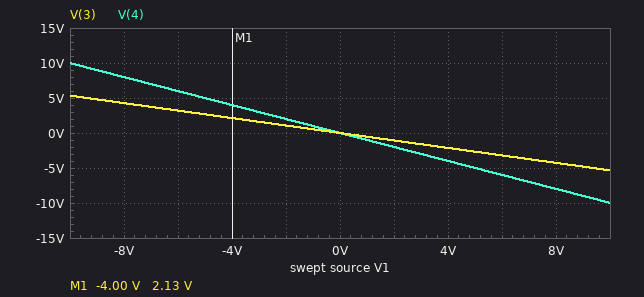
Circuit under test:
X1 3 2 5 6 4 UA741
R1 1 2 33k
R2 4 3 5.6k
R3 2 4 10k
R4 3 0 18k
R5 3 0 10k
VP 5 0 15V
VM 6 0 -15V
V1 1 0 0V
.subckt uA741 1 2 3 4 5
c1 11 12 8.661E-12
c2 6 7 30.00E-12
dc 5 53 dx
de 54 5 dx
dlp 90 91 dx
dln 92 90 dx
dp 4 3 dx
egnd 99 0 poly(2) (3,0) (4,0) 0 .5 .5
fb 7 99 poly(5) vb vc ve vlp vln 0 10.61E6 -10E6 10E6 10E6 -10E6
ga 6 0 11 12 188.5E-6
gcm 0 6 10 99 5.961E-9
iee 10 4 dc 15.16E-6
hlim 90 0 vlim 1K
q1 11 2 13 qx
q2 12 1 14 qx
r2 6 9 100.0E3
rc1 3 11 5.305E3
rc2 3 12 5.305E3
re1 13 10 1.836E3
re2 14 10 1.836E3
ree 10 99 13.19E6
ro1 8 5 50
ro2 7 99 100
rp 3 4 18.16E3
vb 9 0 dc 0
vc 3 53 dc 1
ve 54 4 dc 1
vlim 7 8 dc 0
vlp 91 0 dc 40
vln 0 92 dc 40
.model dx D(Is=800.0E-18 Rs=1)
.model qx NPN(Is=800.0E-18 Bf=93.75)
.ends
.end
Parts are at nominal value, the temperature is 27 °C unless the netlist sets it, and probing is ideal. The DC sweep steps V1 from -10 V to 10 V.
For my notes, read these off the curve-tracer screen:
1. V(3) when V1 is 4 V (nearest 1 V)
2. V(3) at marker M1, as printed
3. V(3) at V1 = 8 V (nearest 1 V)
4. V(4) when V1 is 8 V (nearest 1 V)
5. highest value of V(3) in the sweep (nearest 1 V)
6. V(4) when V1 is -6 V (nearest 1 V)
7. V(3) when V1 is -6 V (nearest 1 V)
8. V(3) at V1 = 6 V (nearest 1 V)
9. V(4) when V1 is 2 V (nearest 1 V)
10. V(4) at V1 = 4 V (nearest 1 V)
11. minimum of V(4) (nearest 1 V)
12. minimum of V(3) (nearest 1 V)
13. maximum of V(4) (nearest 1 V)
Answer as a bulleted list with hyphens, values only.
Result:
- -2 V
- 2.13 V
- -4 V
- -8 V
- 5 V
- 6 V
- 3 V
- -3 V
- -2 V
- -4 V
- -10 V
- -5 V
- 10 V
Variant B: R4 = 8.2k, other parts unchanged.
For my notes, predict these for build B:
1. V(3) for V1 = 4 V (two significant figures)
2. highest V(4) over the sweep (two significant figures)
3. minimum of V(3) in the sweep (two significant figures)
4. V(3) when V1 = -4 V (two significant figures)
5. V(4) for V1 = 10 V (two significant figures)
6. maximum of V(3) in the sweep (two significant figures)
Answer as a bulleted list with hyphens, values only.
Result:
- -1.3 V
- 7.2 V
- -3.2 V
- 1.3 V
- -7.2 V
- 3.2 V
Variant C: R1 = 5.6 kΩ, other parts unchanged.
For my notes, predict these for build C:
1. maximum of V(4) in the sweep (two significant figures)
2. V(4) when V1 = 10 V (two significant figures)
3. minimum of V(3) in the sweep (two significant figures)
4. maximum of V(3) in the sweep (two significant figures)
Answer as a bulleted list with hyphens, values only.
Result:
- 15 V
- -15 V
- -7.8 V
- 7.8 V
